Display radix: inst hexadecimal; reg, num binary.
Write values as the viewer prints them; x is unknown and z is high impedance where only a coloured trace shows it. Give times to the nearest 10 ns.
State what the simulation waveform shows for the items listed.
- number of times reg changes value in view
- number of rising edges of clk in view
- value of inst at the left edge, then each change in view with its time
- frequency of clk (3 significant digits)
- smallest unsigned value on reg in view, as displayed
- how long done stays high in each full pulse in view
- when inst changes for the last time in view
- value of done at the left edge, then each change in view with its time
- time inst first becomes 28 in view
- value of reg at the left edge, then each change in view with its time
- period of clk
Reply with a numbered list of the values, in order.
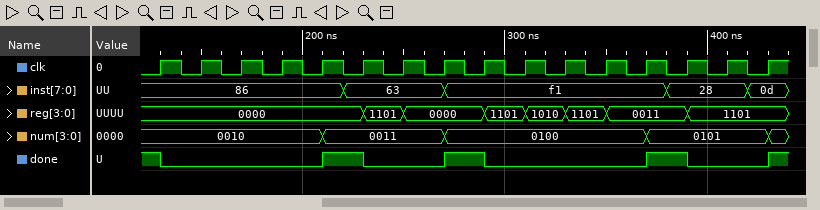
1. 7
2. 16
3. 86, 63 at 220 ns, f1 at 270 ns, 28 at 380 ns, 0d at 420 ns
4. 50.0 MHz
5. 0000
6. 20 ns, 20 ns, 20 ns
7. 420 ns
8. 1, 0 at 130 ns, 1 at 210 ns, 0 at 230 ns, 1 at 270 ns, 0 at 290 ns, 1 at 370 ns, 0 at 390 ns, 1 at 430 ns
9. 380 ns
10. 0000, 1101 at 230 ns, 0000 at 250 ns, 1101 at 290 ns, 1010 at 310 ns, 1101 at 330 ns, 0011 at 350 ns, 1101 at 390 ns
11. 20 ns
